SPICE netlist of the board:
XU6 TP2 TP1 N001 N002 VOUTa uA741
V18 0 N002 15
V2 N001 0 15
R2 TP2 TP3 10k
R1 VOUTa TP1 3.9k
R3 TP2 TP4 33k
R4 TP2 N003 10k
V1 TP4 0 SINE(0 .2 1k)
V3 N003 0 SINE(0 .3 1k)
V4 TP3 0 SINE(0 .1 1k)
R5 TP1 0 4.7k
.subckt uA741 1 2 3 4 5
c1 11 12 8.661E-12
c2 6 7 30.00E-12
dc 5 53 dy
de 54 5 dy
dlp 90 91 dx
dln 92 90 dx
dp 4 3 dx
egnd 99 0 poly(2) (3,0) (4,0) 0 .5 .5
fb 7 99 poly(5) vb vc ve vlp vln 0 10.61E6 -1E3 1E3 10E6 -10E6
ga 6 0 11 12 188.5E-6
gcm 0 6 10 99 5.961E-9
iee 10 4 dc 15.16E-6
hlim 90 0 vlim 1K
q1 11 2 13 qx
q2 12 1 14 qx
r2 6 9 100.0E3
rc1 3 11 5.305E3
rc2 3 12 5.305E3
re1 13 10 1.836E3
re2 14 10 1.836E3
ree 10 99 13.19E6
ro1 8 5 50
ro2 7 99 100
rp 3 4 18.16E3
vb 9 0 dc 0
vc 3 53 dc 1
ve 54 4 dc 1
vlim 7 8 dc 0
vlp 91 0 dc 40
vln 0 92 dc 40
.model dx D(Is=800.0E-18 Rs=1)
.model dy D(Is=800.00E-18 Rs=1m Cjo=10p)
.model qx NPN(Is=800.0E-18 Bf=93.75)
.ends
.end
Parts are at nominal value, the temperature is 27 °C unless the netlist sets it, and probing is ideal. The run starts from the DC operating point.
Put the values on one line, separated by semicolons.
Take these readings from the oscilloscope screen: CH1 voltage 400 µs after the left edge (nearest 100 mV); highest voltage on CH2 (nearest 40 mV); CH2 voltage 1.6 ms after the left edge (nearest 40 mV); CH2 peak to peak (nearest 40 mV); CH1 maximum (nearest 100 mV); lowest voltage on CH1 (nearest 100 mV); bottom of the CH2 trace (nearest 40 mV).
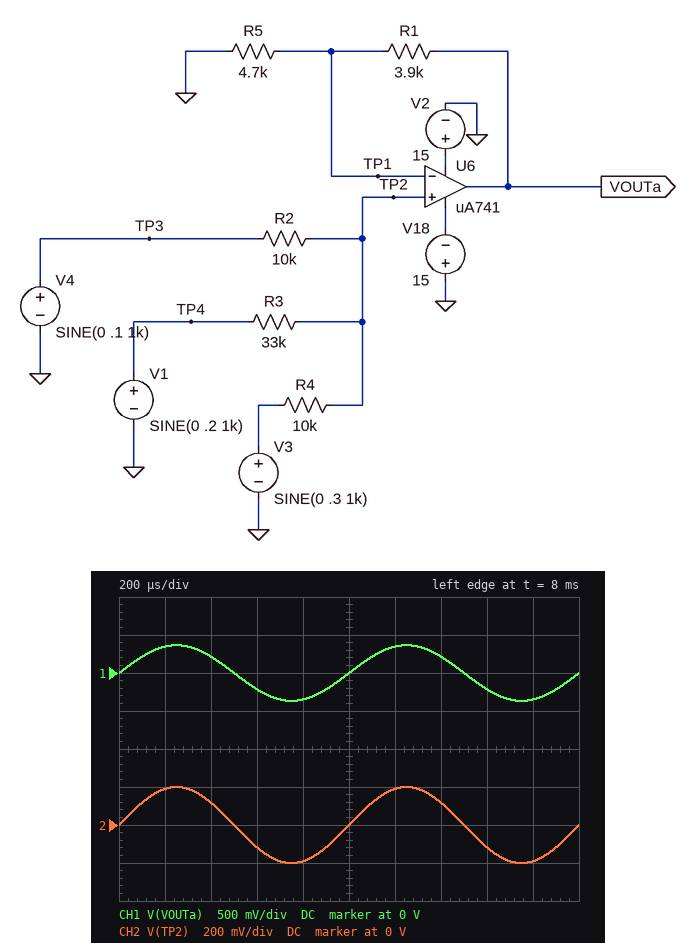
200 mV; 200 mV; -120 mV; 400 mV; 400 mV; -400 mV; -200 mV
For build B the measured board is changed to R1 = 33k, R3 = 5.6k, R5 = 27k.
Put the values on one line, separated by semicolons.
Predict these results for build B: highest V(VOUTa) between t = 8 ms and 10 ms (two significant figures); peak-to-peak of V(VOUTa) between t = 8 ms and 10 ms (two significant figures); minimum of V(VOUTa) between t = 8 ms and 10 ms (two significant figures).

450 mV; 890 mV; -440 mV
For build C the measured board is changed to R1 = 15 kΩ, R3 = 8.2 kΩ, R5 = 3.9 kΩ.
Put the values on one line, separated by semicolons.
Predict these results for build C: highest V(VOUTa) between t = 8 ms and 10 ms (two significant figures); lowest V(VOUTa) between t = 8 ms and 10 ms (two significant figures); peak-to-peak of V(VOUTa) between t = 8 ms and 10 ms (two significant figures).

970 mV; -970 mV; 1.9 V
